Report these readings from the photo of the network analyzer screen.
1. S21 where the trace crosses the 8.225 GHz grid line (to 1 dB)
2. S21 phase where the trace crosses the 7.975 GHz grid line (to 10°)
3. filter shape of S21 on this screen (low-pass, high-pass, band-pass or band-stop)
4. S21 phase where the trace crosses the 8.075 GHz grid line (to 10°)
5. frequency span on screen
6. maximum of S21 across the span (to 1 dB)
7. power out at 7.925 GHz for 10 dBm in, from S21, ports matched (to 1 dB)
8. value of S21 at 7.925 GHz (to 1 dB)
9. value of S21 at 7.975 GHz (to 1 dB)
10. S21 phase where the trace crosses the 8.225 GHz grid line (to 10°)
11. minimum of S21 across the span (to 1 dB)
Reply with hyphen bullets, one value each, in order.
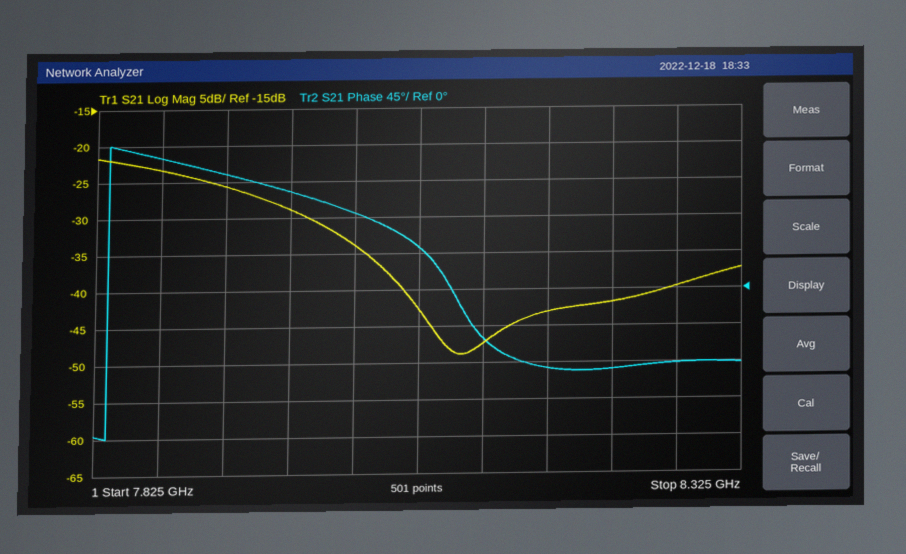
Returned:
- -42 dB
- 120°
- low-pass
- 50°
- 500 MHz
- -22 dB
- -16 dBm
- -26 dB
- -29 dB
- -100°
- -49 dB
